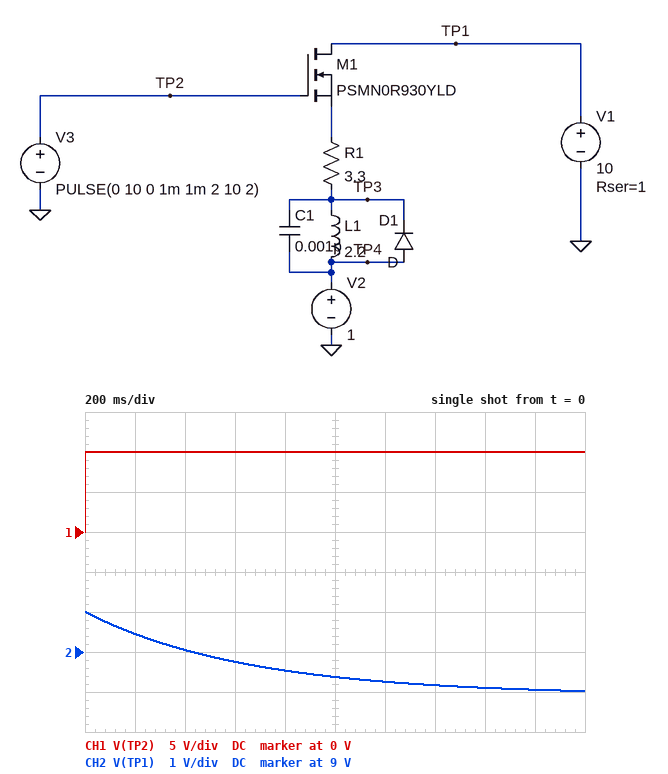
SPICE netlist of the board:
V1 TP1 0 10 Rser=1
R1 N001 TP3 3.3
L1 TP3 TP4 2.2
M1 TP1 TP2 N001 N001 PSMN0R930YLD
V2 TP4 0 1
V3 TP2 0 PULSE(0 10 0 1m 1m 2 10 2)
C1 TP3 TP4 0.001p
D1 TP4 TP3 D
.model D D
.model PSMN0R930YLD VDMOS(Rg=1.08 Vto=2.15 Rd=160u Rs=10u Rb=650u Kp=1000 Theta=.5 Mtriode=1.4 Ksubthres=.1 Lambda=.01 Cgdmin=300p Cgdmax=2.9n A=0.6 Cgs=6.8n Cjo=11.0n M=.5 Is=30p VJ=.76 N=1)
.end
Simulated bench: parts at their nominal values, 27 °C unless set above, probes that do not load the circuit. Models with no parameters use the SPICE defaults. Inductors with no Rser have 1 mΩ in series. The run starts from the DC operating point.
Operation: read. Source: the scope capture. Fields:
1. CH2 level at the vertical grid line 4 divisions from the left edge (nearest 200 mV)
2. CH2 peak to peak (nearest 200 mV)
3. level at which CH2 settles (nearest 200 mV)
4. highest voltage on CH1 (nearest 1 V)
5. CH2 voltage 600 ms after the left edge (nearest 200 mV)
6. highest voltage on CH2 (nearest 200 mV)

8.6 V
2.0 V
8.0 V
10 V
8.8 V
10.0 V
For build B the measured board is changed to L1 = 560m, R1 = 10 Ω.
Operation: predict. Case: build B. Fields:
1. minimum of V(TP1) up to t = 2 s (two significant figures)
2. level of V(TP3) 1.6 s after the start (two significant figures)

9.3 V
1.0 V
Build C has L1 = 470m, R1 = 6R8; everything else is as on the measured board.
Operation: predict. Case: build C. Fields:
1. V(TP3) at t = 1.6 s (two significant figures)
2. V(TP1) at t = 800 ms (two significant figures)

1.0 V
9.0 V
